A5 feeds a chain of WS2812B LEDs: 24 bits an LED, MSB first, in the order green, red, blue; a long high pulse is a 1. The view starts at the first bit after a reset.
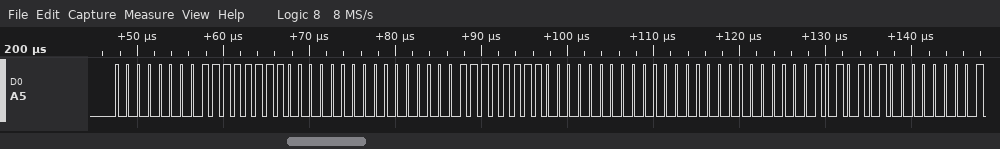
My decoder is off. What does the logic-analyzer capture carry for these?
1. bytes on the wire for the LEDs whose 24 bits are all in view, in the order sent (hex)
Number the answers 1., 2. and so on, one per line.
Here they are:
1. 00 FF 00 00 FF 00 00 00 55
